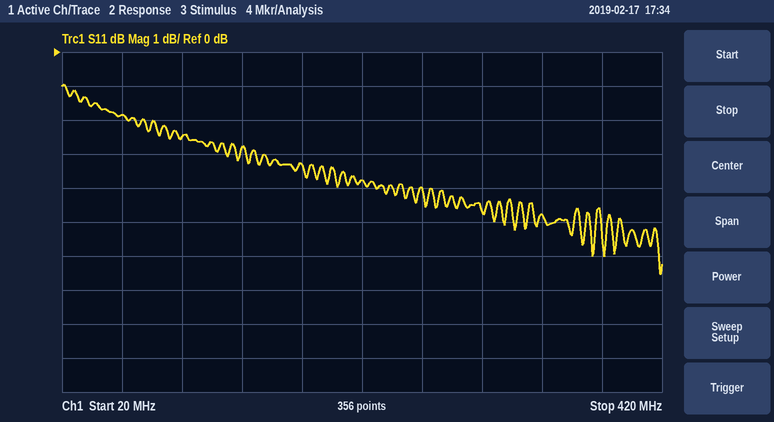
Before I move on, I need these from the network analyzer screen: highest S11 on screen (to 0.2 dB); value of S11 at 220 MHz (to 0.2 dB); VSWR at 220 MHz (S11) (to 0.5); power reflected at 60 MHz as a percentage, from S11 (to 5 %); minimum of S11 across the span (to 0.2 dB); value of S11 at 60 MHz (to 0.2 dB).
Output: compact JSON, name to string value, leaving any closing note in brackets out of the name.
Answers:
{"highest S11 on screen": "-1.0 dB", "value of S11 at 220 MHz": "-3.8 dB", "VSWR at 220 MHz (S11)": "4.5", "power reflected at 60 MHz as a percentage, from S11": "65 %", "minimum of S11 across the span": "-6.6 dB", "value of S11 at 60 MHz": "-1.8 dB"}
